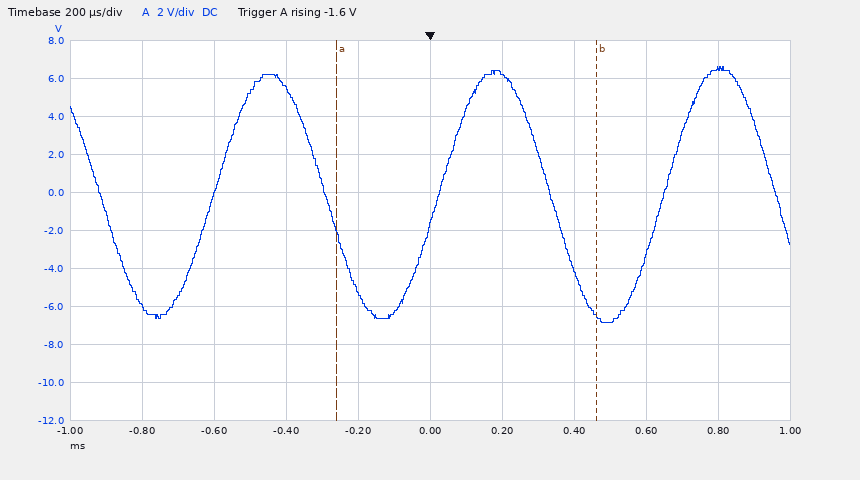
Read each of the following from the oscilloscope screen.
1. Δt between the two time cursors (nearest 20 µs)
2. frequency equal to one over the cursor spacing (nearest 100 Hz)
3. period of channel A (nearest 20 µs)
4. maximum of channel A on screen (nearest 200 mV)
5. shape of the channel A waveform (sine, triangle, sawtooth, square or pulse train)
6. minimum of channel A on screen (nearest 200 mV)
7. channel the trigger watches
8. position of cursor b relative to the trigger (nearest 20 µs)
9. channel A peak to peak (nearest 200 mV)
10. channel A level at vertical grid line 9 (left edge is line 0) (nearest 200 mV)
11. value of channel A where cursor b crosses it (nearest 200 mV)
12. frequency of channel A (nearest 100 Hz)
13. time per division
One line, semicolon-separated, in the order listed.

720 µs; 1.4 kHz; 620 µs; 6.6 V; sine; -6.8 V; channel A; +460 µs; 13.4 V; 6.6 V; -6.4 V; 1.6 kHz; 200 µs
